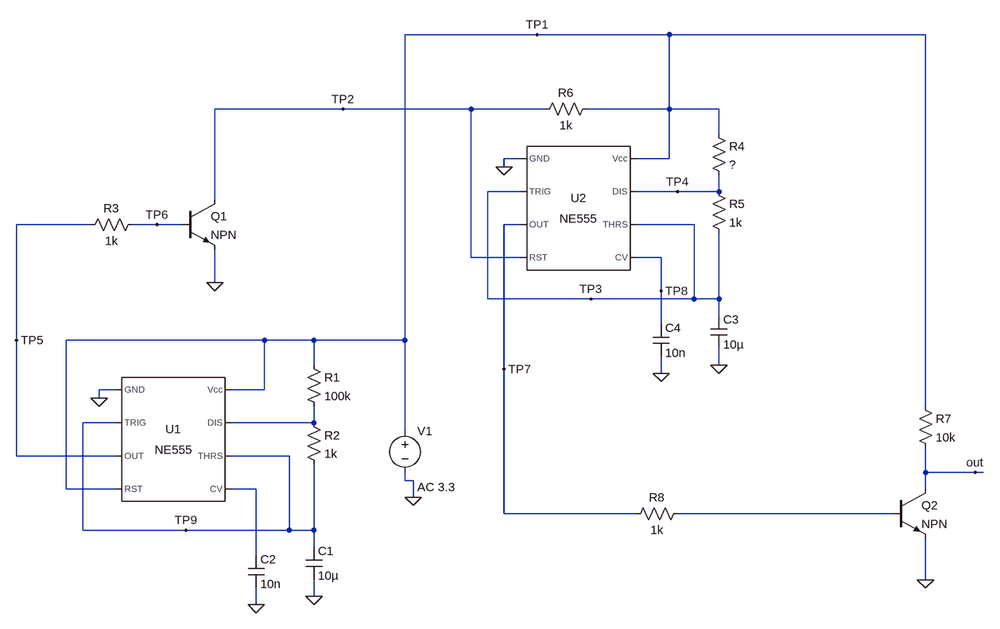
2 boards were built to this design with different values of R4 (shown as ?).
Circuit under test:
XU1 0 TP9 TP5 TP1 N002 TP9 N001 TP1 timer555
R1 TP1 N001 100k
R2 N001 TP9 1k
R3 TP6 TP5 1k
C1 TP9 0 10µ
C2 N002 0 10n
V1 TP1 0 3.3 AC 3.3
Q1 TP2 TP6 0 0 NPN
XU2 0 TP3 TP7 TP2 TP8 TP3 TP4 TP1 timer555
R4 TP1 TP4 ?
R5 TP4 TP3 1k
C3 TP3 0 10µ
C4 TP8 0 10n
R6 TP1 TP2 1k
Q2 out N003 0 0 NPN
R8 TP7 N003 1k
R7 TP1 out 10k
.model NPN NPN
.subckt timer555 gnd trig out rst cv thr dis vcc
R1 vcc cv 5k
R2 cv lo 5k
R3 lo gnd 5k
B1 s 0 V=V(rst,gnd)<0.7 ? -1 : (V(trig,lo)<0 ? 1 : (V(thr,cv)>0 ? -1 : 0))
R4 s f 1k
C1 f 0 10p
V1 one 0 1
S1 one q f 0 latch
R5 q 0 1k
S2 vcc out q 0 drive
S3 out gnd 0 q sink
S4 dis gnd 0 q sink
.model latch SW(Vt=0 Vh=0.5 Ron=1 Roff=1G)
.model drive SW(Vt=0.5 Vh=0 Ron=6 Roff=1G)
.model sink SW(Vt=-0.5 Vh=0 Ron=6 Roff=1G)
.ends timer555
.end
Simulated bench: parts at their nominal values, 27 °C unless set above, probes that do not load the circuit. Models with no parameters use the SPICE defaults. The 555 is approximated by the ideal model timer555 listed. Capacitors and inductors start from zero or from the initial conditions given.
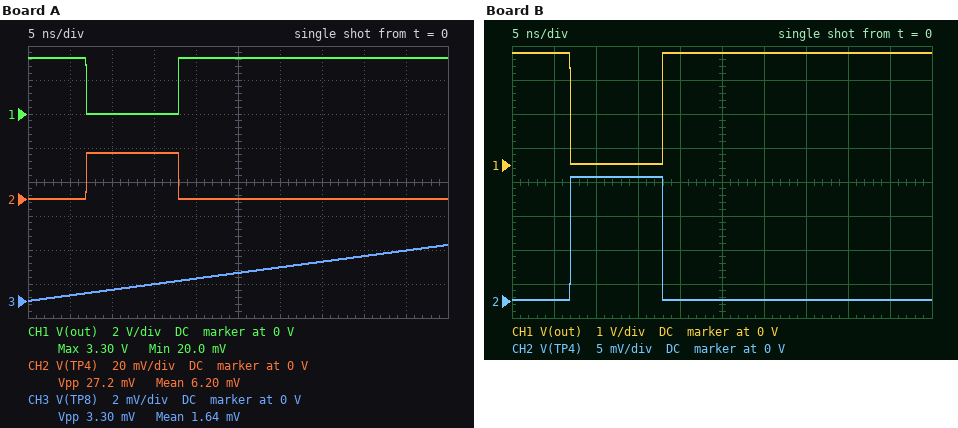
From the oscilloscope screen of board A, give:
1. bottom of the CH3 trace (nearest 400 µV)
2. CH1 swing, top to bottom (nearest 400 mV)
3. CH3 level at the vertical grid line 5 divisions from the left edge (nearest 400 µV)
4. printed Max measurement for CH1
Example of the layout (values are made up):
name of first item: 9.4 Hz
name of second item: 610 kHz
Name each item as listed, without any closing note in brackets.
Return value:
bottom of the CH3 trace: 0 V
CH1 swing, top to bottom: 3.2 V
CH3 level at the vertical grid line 5 divisions from the left edge: 1.6 mV
printed Max measurement for CH1: 3.30 V
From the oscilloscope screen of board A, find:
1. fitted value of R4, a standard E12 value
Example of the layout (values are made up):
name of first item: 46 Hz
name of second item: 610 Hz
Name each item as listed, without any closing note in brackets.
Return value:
fitted value of R4, a standard E12 value: 120 kΩ
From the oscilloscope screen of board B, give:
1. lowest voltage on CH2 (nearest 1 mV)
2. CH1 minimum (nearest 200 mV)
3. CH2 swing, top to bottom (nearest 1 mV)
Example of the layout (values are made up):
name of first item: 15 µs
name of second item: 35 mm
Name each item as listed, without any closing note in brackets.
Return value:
lowest voltage on CH2: 0 V
CH1 minimum: 0 V
CH2 swing, top to bottom: 18 mV
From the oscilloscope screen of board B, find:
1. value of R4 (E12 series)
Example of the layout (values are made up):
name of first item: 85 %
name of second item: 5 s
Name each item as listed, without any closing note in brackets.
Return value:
value of R4: 180 kΩ
